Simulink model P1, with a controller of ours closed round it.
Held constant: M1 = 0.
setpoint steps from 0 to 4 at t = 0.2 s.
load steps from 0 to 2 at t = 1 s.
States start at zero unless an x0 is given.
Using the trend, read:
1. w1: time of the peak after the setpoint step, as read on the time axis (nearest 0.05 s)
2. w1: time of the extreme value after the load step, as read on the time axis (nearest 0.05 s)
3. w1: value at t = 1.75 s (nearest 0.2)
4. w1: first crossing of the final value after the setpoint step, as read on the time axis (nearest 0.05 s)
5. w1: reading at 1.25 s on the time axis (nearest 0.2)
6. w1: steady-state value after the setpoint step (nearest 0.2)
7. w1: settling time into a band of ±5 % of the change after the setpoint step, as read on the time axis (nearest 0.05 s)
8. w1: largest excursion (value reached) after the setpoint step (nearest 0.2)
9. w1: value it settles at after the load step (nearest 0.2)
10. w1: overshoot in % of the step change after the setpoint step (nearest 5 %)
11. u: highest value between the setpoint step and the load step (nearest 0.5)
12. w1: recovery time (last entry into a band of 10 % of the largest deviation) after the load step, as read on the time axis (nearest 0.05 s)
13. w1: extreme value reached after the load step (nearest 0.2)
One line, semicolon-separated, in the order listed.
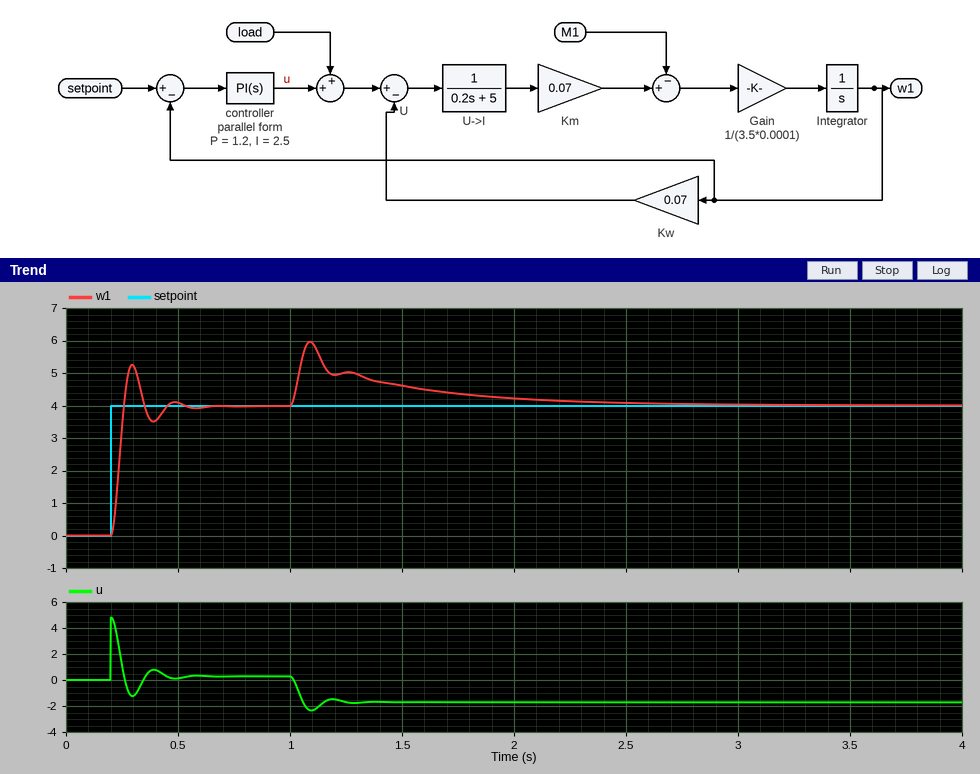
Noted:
0.30 s; 1.10 s; 4.4; 0.25 s; 5.0; 4.0; 0.45 s; 5.2; 4.0; 30 %; 5.0; 2.05 s; 6.0
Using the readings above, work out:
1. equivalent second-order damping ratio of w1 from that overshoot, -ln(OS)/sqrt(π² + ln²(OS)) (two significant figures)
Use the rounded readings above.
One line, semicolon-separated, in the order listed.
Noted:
0.36
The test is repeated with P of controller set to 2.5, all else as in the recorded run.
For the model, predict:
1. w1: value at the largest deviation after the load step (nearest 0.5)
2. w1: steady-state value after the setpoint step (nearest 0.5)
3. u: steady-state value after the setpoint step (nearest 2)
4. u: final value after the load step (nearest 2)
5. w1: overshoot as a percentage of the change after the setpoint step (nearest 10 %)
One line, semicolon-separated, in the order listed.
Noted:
5.0; 4.0; 0; -2; 40 %
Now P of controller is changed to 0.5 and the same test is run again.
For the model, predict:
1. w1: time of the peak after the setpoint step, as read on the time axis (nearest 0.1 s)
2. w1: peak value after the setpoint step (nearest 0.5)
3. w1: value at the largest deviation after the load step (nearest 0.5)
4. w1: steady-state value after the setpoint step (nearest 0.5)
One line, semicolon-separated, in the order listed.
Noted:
0.4 s; 5.0; 7.5; 4.0
